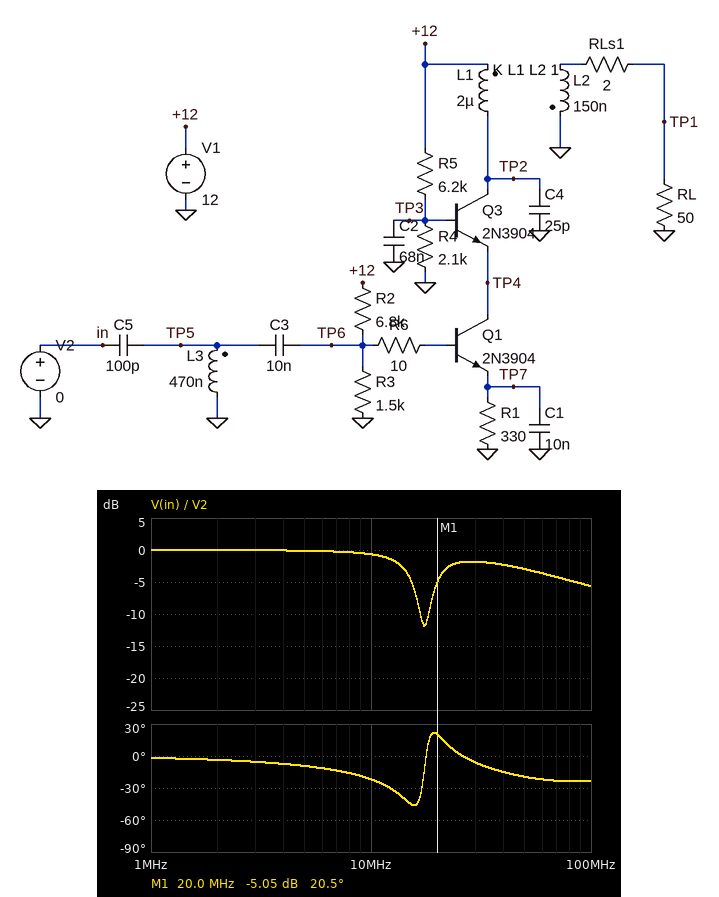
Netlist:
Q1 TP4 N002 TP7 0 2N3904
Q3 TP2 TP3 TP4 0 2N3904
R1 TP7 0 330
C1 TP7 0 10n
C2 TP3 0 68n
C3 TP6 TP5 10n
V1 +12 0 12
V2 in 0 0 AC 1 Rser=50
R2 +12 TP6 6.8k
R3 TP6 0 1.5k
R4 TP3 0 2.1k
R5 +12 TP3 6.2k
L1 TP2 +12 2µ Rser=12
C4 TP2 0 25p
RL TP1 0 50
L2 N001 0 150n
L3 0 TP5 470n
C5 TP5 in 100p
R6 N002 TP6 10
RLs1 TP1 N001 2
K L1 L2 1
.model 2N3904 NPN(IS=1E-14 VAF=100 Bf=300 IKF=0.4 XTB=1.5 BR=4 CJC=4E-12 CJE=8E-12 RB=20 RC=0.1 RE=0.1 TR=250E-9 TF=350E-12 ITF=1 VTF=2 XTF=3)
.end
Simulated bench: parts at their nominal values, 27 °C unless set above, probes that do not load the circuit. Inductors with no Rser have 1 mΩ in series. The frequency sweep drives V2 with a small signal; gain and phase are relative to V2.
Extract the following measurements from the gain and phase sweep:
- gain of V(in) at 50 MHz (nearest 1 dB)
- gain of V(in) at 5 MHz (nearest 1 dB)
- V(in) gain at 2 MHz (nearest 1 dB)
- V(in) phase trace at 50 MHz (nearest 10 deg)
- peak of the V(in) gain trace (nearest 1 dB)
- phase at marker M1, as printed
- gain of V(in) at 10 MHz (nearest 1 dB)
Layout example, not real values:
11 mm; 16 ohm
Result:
-3 dB; 0 dB; 0 dB; -20 deg; 0 dB; 20.5 deg; -1 dB
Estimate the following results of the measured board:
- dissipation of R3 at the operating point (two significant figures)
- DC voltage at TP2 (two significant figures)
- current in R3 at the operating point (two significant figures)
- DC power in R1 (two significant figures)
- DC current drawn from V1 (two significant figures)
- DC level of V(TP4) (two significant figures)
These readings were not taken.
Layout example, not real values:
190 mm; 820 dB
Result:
3.1 mW; 12 V; 1.4 mA; 6.4 mW; 7.3 mA; 2.3 V
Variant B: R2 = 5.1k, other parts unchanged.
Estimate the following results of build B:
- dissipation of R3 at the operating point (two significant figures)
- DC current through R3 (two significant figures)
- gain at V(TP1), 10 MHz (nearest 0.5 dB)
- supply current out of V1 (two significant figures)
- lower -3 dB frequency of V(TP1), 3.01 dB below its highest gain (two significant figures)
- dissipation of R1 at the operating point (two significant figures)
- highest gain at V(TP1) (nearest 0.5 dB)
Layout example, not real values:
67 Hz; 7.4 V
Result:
4.9 mW; 1.8 mA; 7.5 dB; 9.3 mA; 16 MHz; 12 mW; 31.0 dB
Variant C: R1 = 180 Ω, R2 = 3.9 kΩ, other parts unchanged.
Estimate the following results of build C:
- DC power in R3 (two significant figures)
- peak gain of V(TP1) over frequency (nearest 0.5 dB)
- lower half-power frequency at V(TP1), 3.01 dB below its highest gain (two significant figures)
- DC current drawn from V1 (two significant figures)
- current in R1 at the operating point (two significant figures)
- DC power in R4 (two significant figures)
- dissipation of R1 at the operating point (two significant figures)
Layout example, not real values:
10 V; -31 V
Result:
5.7 mW; -4.5 dB; 16 MHz; 16 mA; 12 mA; 4.2 mW; 27 mW
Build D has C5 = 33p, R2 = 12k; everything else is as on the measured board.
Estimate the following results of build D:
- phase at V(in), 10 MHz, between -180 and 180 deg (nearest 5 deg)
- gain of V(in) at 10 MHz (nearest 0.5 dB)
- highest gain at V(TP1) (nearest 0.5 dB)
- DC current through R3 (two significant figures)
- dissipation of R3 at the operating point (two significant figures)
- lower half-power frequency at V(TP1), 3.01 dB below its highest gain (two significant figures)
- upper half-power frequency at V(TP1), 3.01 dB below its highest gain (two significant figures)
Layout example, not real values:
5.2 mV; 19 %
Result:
-5 deg; 0 dB; 22.5 dB; 880 µA; 1.2 mW; 22 MHz; 29 MHz
